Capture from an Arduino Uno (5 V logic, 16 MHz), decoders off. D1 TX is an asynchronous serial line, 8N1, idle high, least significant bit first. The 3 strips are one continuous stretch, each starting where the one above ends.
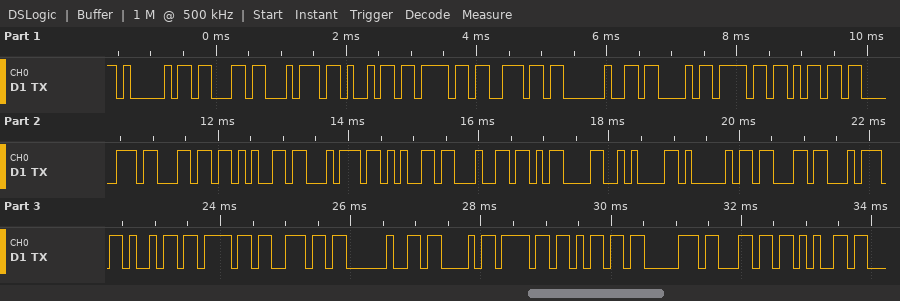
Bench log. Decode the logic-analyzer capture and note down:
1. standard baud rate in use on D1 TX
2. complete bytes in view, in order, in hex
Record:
9600 baud
41 63 74 69 6F 6E 20 43 6F 6D 70 6C 65 74 65 64 0D 0A 41 63 74 69 6F 6E 20 43 6F 6D 70 6C 65
